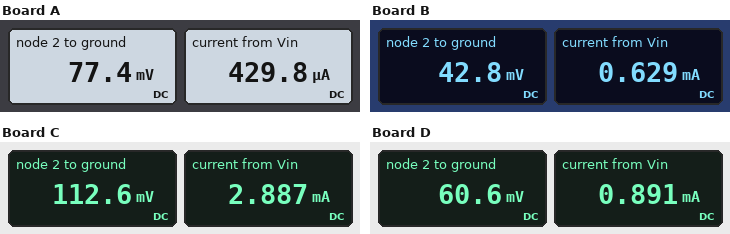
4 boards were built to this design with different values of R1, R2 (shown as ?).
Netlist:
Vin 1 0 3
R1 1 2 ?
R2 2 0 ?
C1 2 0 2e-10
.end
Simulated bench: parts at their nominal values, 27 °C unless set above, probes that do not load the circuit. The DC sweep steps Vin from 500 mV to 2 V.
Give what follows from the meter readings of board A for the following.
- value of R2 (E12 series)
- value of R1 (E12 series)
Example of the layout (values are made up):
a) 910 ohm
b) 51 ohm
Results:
a) 180 Ω
b) 6.8 kΩ
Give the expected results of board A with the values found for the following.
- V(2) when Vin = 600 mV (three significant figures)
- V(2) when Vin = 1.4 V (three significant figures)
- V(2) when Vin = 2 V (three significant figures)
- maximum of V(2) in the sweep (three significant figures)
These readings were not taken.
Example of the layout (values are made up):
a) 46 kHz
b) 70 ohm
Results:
a) 15.5 mV
b) 36.1 mV
c) 51.6 mV
d) 51.6 mV
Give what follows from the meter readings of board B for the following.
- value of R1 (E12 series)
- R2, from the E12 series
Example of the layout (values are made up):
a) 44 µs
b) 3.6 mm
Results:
a) 4.7 kΩ
b) 68 Ω
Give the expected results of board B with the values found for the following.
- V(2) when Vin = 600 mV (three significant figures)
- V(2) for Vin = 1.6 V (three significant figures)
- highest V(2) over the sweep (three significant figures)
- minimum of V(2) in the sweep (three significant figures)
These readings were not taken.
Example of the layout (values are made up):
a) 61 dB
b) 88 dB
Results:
a) 8.56 mV
b) 22.8 mV
c) 28.5 mV
d) 7.13 mV
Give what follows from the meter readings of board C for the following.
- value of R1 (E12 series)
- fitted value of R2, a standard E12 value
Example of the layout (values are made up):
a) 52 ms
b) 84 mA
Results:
a) 1 kΩ
b) 39 Ω
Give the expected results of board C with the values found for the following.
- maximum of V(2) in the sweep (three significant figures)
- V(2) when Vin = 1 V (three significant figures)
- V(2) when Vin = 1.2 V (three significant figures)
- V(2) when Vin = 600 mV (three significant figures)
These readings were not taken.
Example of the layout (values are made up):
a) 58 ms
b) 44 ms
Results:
a) 75.1 mV
b) 37.5 mV
c) 45.0 mV
d) 22.5 mV
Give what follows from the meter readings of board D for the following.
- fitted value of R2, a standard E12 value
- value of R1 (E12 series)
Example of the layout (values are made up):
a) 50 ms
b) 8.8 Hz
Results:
a) 68 Ω
b) 3.3 kΩ
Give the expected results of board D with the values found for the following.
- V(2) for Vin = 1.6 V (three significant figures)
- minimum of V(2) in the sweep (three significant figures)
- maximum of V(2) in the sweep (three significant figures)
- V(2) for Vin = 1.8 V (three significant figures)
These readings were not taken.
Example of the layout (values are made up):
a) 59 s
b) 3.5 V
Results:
a) 32.3 mV
b) 10.1 mV
c) 40.4 mV
d) 36.3 mV
